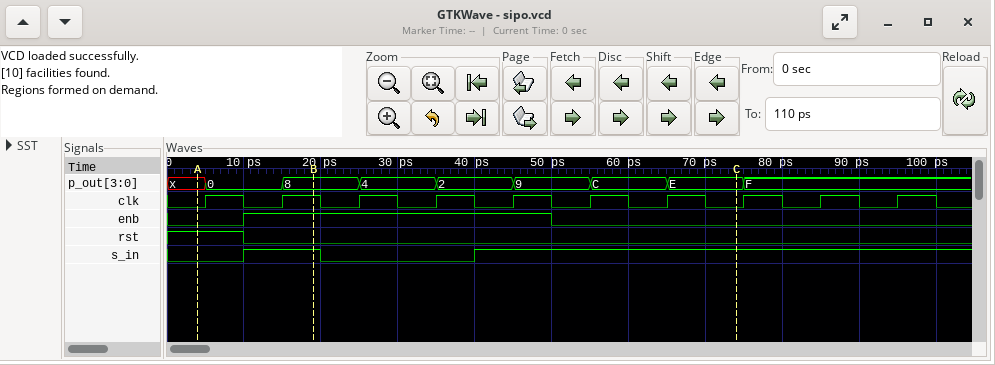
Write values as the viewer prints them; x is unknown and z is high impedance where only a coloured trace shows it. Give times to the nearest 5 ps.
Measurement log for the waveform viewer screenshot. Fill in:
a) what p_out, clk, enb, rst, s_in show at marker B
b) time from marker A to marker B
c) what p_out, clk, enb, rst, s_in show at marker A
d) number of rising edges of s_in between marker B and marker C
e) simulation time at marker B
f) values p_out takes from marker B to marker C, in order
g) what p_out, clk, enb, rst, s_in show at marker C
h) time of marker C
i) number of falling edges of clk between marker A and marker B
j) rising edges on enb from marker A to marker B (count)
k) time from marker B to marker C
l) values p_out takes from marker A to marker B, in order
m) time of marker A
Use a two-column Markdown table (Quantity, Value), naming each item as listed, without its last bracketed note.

| Quantity | Value |
|---|---|
| what p_out, clk, enb, rst, s_in show at marker B | p_out=8, clk=1, enb=1, rst=0, s_in=1 |
| time from marker A to marker B | 15 ps |
| what p_out, clk, enb, rst, s_in show at marker A | p_out=x, clk=0, enb=0, rst=1, s_in=0 |
| number of rising edges of s_in between marker B and marker C | 1 |
| simulation time at marker B | 20 ps |
| values p_out takes from marker B to marker C, in order | 8, 4, 2, 9, C, E |
| what p_out, clk, enb, rst, s_in show at marker C | p_out=E, clk=0, enb=0, rst=0, s_in=1 |
| time of marker C | 75 ps |
| number of falling edges of clk between marker A and marker B | 1 |
| rising edges on enb from marker A to marker B | 1 |
| time from marker B to marker C | 55 ps |
| values p_out takes from marker A to marker B, in order | x, 0, 8 |
| time of marker A | 5 ps |
